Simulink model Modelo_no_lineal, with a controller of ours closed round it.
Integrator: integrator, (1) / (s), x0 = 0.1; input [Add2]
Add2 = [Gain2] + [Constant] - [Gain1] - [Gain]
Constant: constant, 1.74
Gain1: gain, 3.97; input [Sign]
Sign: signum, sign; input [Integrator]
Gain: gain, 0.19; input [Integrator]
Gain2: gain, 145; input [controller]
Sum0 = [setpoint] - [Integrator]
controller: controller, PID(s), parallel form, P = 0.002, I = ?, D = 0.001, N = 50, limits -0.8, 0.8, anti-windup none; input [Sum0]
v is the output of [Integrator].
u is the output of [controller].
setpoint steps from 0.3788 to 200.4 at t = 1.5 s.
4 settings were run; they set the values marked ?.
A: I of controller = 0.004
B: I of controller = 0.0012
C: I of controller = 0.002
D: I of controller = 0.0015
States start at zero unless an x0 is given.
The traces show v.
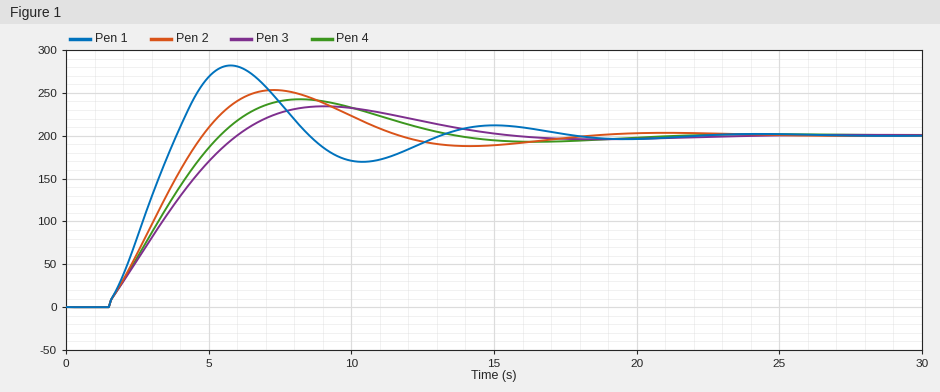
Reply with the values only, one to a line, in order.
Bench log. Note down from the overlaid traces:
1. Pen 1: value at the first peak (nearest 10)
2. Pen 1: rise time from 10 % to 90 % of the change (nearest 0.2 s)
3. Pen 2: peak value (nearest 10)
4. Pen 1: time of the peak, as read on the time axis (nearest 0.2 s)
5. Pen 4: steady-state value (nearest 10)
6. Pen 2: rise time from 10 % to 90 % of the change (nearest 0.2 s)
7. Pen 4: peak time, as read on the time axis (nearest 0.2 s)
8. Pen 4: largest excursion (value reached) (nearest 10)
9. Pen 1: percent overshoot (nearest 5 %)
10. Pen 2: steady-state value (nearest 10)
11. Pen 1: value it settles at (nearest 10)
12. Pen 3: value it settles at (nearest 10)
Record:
280
1.8 s
250
5.8 s
200
2.6 s
8.2 s
240
40 %
200
200
200
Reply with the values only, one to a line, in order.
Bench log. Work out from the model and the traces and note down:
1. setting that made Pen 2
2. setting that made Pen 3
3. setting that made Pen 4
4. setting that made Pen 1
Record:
C
B
D
A
